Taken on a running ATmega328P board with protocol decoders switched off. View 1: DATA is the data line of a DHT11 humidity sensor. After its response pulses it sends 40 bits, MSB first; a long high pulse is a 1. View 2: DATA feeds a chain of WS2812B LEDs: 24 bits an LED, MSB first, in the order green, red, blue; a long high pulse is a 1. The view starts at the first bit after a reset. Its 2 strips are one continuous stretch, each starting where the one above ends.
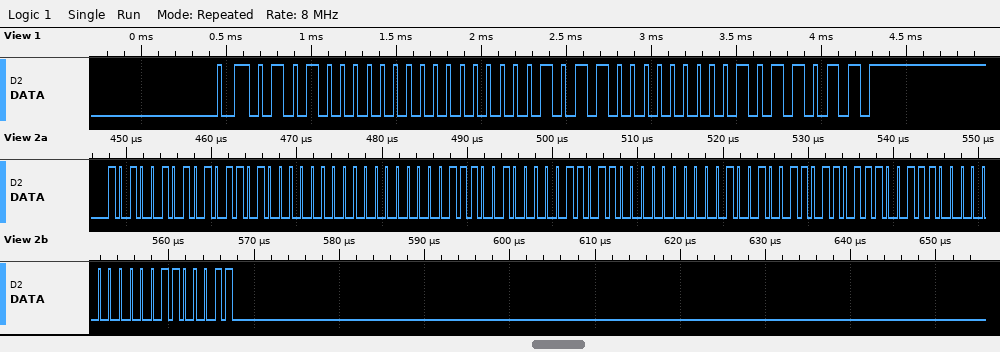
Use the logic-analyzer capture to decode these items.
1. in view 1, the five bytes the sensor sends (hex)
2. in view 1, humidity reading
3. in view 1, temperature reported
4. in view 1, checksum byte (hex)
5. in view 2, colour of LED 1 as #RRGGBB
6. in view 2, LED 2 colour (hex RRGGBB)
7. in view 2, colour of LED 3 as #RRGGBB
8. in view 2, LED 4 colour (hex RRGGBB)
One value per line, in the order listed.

50 00 0B 00 5B
80 %
11.0 °C
0x5B
#5AA500
#E4001B
#2400DB
#009C63
